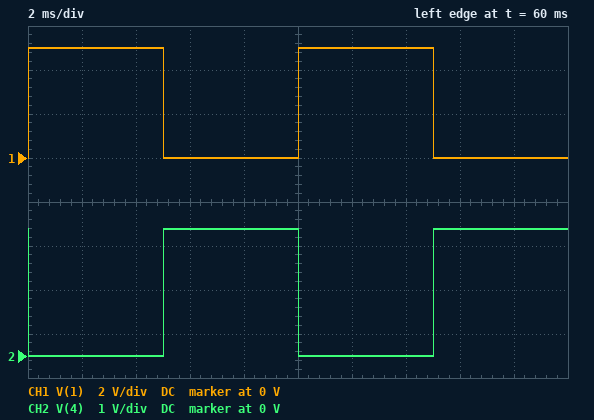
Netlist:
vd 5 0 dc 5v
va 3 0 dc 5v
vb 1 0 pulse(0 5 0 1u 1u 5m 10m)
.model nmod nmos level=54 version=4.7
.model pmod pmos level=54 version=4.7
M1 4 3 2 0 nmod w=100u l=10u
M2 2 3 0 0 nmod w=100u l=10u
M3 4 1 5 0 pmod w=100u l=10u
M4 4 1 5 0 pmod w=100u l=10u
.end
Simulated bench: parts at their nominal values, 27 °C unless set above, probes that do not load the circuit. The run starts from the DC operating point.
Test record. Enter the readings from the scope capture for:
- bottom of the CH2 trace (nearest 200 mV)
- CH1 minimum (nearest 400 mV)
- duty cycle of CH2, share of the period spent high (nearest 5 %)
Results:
0 V
0 V
50 %
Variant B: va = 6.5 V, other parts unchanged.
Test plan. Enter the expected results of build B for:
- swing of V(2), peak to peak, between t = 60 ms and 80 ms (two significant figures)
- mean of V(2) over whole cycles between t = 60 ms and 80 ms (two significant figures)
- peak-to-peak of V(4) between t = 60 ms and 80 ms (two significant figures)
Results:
1.1 V
560 mV
2.4 V
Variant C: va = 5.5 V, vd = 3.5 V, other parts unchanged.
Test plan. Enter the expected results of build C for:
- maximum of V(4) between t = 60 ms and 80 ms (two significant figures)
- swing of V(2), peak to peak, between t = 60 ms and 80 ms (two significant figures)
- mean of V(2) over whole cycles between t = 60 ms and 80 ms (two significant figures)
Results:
1.5 V
720 mV
360 mV
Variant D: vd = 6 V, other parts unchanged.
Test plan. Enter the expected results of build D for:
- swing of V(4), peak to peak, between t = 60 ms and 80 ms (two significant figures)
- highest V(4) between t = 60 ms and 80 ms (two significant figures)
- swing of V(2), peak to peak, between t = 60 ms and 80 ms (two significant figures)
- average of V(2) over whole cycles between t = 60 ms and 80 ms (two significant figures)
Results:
3.6 V
3.9 V
1.3 V
800 mV
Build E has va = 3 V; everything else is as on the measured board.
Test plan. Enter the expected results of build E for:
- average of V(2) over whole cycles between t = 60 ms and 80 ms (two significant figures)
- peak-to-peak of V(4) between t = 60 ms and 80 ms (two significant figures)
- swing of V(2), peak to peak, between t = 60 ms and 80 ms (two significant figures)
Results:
430 mV
4.2 V
850 mV
